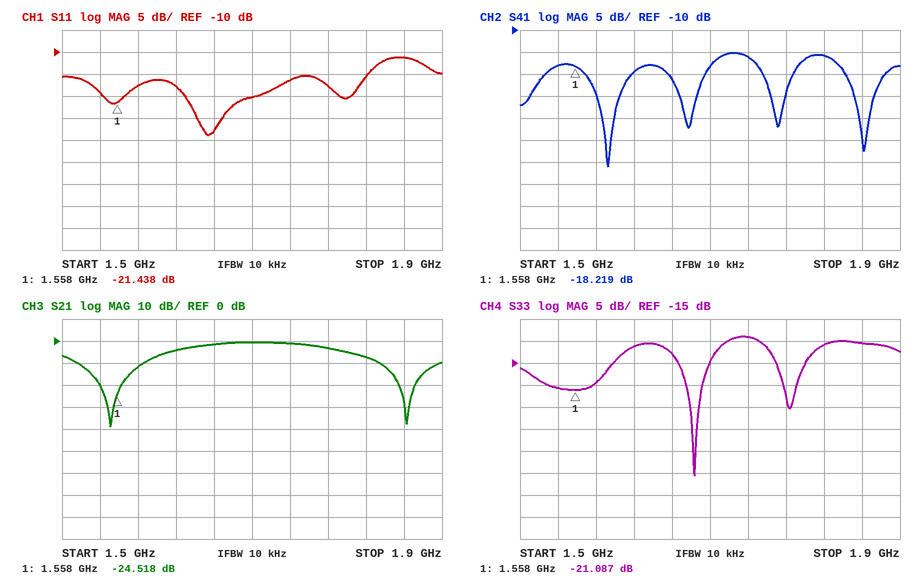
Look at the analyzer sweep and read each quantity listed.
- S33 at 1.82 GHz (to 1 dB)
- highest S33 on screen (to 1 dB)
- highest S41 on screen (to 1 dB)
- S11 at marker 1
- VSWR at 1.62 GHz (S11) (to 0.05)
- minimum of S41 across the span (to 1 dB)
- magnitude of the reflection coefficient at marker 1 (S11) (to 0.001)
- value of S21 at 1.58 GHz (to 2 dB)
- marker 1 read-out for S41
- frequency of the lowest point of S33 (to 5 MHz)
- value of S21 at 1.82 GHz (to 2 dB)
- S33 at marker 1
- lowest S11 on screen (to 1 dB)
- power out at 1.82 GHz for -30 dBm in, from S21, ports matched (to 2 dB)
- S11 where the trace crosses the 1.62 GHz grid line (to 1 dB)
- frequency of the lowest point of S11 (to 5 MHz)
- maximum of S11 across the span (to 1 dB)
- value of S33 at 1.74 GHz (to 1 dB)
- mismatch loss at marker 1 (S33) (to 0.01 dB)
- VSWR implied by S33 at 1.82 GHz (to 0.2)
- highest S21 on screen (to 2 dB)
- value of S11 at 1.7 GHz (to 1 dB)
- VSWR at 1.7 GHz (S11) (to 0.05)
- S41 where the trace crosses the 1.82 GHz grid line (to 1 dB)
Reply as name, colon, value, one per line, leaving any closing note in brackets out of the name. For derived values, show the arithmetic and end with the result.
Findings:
S33 at 1.82 GHz: -11 dB
highest S33 on screen: -9 dB
highest S41 on screen: -15 dB
S11 at marker 1: -21.438 dB
VSWR at 1.62 GHz (S11): |Γ| = 10^(-18/20) = 0.1259; VSWR = (1 + 0.1259)/(1 − 0.1259) ≈ 1.29, so 1.30 to the nearest 0.05
minimum of S41 across the span: -41 dB
magnitude of the reflection coefficient at marker 1 (S11): 10^(-21.438/20) ≈ 0.085
value of S21 at 1.58 GHz: -12 dB
marker 1 read-out for S41: -18.219 dB
frequency of the lowest point of S33: 1.685 GHz
value of S21 at 1.82 GHz: -8 dB
S33 at marker 1: -21.087 dB
lowest S11 on screen: -29 dB
power out at 1.82 GHz for -30 dBm in, from S21, ports matched: -30 dBm + (-8 dB) = -38 dBm
S11 where the trace crosses the 1.62 GHz grid line: -18 dB
frequency of the lowest point of S11: 1.655 GHz
maximum of S11 across the span: -11 dB
value of S33 at 1.74 GHz: -9 dB
mismatch loss at marker 1 (S33): −10 log10(1 − 10^(-21.087/10)) ≈ 0.03 dB
VSWR implied by S33 at 1.82 GHz: |Γ| = 10^(-11/20) = 0.2818; VSWR = (1 + 0.2818)/(1 − 0.2818) ≈ 1.8
highest S21 on screen: 0 dB
value of S11 at 1.7 GHz: -20 dB
VSWR at 1.7 GHz (S11): |Γ| = 10^(-20/20) = 0.1000; VSWR = (1 + 0.1000)/(1 − 0.1000) ≈ 1.22, so 1.20 to the nearest 0.05
S41 where the trace crosses the 1.82 GHz grid line: -16 dB
